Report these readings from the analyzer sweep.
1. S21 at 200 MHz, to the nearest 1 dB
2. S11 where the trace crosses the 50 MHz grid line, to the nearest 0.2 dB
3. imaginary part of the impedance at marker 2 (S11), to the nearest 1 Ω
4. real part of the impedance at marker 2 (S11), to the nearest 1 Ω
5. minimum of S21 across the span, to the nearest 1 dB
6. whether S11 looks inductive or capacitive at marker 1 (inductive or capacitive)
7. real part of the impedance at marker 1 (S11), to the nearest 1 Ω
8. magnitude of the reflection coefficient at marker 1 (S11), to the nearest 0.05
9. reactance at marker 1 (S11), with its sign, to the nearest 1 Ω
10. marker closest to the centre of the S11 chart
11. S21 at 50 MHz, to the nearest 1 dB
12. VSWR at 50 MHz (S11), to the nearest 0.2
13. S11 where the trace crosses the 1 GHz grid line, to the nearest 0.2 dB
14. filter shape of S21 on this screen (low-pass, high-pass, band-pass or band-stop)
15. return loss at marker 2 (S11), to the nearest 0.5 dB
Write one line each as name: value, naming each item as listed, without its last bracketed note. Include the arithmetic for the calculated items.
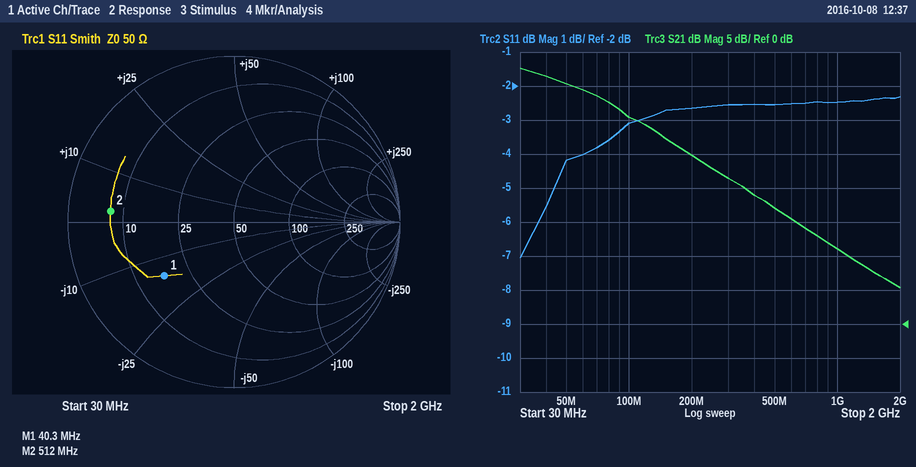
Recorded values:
S21 at 200 MHz, to the nearest 1 dB: 25 dB
S11 where the trace crosses the 50 MHz grid line, to the nearest 0.2 dB: -4.2 dB
imaginary part of the impedance at marker 2 (S11), to the nearest 1 Ω: +2 Ω
real part of the impedance at marker 2 (S11), to the nearest 1 Ω: 7 Ω
minimum of S21 across the span, to the nearest 1 dB: 5 dB
whether S11 looks inductive or capacitive at marker 1: capacitive
real part of the impedance at marker 1 (S11), to the nearest 1 Ω: 17 Ω
magnitude of the reflection coefficient at marker 1 (S11), to the nearest 0.05: 0.55
reactance at marker 1 (S11), with its sign, to the nearest 1 Ω: -15 Ω
marker closest to the centre of the S11 chart: marker 1
S21 at 50 MHz, to the nearest 1 dB: 35 dB
VSWR at 50 MHz (S11), to the nearest 0.2: |Γ| = 10^(-4.2/20) = 0.6166; VSWR = (1 + 0.6166)/(1 − 0.6166) ≈ 4.2
S11 where the trace crosses the 1 GHz grid line, to the nearest 0.2 dB: -2.4 dB
filter shape of S21 on this screen: low-pass
return loss at marker 2 (S11), to the nearest 0.5 dB: 2.5 dB
